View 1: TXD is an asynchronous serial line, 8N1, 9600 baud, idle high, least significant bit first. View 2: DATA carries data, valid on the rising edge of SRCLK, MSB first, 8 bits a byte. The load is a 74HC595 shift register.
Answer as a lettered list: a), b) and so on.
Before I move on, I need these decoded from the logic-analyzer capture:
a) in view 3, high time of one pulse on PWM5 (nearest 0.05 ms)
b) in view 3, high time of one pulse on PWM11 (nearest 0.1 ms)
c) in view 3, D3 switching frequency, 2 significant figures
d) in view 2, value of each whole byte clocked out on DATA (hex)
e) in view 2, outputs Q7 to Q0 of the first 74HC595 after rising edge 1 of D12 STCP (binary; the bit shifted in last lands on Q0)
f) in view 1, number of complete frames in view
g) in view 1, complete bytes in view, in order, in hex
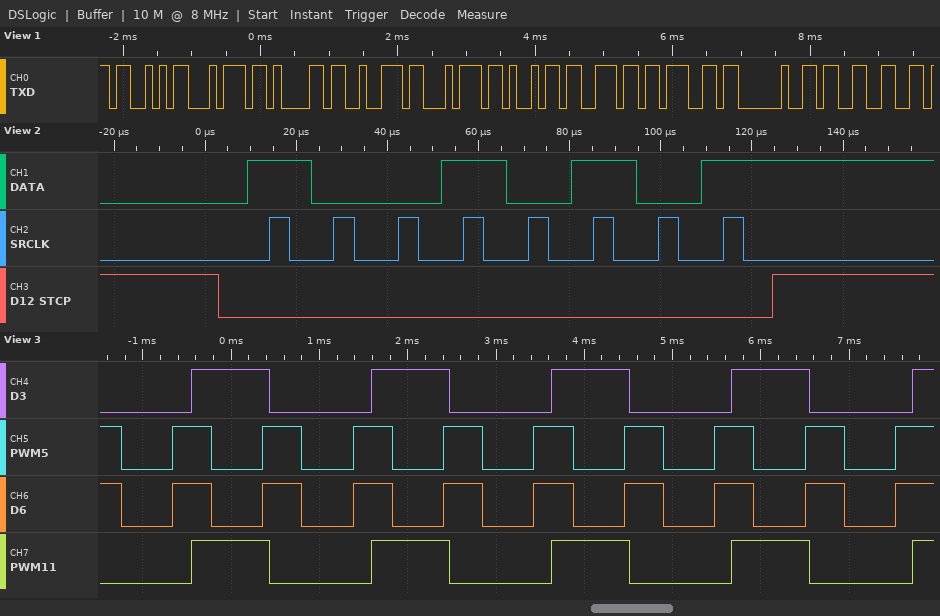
a) 0.45 ms
b) 0.9 ms
c) 490 Hz
d) 95
e) 10010101
f) 10
g) 53 74 61 72 74 69 6E 67 20 33
